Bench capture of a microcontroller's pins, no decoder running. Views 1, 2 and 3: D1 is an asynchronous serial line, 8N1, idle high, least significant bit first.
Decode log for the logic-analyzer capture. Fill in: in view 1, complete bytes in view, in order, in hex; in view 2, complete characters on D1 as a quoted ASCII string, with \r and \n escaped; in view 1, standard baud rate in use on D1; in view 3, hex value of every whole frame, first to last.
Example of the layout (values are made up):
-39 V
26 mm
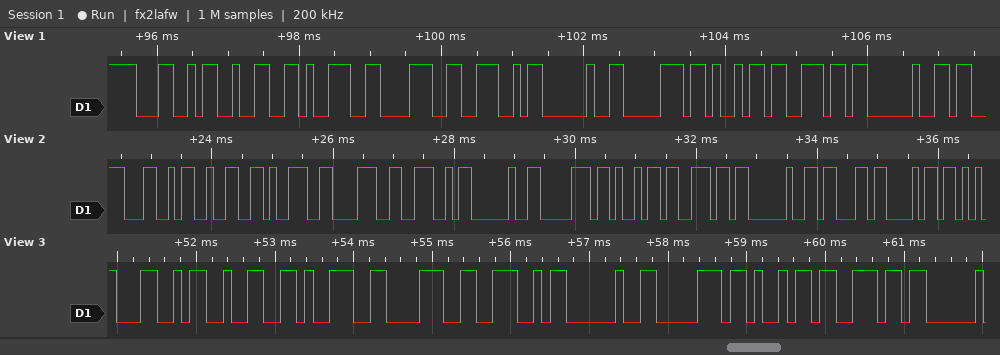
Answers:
0x4C 0x32 0x39 0x38 0x4E 0x20 0x70 0x69 0x6E 0x20
"L298N pin ch"
9600 baud
4C 32 39 38 4E 20 70 69 6E
